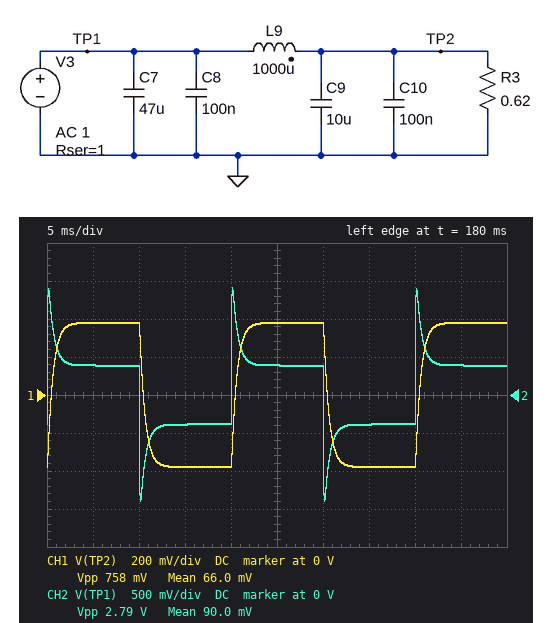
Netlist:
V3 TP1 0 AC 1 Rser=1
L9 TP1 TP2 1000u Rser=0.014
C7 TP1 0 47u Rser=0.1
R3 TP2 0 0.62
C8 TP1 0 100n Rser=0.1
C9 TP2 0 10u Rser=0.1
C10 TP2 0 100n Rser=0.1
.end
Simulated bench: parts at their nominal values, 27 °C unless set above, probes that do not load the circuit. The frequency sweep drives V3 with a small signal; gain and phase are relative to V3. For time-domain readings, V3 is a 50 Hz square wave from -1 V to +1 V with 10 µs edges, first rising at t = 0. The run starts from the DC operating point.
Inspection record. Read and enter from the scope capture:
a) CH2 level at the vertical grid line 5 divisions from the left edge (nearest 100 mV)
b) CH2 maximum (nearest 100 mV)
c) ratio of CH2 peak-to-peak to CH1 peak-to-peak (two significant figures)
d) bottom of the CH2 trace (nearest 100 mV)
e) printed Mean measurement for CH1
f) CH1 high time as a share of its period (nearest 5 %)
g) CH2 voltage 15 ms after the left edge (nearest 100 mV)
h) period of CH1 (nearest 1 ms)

400 mV
1.4 V
3.7
-1.4 V
66.0 mV
50 %
-400 mV
20 ms
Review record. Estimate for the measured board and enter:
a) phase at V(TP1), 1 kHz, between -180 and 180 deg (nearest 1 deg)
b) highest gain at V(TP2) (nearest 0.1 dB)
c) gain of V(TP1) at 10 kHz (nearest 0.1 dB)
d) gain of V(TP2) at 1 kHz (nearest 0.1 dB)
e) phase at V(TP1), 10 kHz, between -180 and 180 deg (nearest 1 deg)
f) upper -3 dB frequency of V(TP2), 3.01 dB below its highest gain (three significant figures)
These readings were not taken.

-8 deg
-8.4 dB
-10.2 dB
-20.4 dB
-56 deg
273 Hz
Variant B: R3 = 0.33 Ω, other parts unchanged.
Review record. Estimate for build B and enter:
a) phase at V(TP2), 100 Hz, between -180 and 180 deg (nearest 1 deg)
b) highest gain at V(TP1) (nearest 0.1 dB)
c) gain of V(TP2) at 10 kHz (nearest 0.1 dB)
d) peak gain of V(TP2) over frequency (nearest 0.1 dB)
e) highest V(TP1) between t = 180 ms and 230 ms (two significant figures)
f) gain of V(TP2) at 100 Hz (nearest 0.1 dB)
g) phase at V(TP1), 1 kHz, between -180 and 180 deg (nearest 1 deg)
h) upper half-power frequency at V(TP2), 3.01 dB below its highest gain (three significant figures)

-26 deg
-0.2 dB
-56.1 dB
-12.2 dB
1.5 V
-13.0 dB
-8 deg
224 Hz
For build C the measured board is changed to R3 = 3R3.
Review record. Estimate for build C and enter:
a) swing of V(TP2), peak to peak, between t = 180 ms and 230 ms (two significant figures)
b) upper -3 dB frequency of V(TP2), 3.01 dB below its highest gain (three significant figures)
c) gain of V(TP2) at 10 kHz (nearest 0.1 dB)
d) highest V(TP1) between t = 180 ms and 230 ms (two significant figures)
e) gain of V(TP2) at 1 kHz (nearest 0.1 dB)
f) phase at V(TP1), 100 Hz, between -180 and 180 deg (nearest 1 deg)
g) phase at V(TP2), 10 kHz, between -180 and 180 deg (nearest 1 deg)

1.5 V
766 Hz
-43.2 dB
1.0 V
-6.8 dB
1 deg
153 deg
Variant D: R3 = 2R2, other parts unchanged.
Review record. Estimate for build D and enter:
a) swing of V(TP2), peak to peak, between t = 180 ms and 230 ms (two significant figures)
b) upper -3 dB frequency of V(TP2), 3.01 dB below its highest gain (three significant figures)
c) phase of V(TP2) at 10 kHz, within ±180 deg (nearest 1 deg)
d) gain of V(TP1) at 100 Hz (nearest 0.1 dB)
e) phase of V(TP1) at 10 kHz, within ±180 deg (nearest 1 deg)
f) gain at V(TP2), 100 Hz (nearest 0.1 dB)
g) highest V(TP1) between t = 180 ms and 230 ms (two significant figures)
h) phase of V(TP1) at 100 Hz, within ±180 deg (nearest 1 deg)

1.4 V
551 Hz
162 deg
-3.1 dB
-56 deg
-3.4 dB
1.1 V
3 deg
